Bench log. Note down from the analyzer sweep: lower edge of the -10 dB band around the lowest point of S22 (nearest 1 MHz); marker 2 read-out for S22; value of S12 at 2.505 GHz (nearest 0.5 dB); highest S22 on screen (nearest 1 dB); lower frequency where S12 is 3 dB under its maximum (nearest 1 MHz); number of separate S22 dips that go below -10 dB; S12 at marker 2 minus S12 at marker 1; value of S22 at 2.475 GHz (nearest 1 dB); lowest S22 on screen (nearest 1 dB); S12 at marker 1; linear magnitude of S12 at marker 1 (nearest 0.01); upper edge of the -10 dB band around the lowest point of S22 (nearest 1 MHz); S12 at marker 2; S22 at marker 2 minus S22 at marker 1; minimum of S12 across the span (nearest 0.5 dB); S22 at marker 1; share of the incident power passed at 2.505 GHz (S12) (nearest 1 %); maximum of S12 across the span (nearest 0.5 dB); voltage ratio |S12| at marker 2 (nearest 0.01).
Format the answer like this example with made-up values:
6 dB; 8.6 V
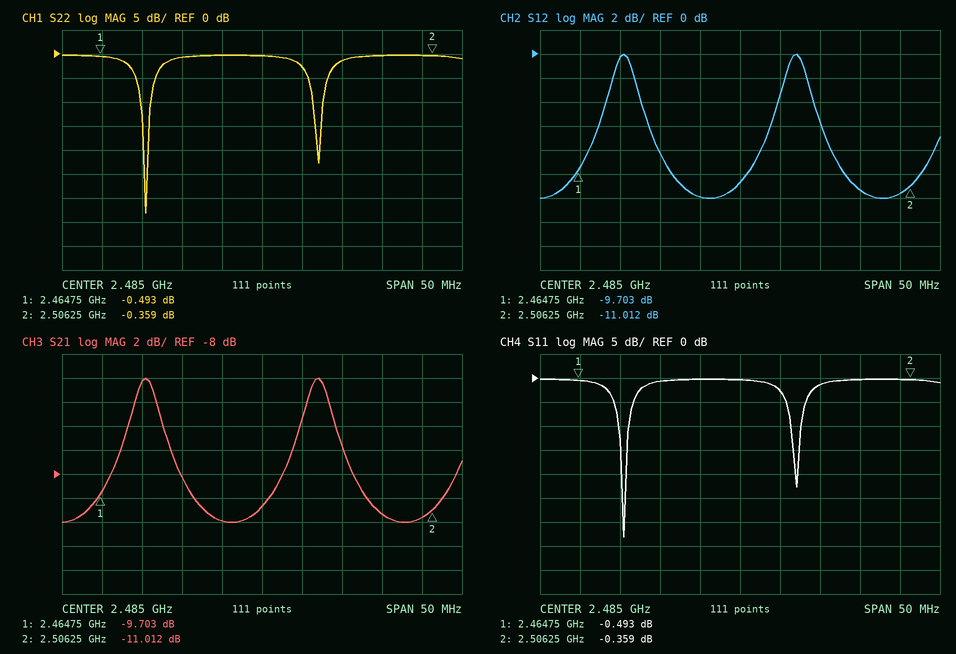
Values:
2.470 GHz; -0.359 dB; -11.5 dB; 0 dB; 2.469 GHz; 2; -1.309 dB; -1 dB; -33 dB; -9.703 dB; 0.33; 2.471 GHz; -11.012 dB; 0.134 dB; -12.0 dB; -0.493 dB; 7 %; 0.0 dB; 0.28
